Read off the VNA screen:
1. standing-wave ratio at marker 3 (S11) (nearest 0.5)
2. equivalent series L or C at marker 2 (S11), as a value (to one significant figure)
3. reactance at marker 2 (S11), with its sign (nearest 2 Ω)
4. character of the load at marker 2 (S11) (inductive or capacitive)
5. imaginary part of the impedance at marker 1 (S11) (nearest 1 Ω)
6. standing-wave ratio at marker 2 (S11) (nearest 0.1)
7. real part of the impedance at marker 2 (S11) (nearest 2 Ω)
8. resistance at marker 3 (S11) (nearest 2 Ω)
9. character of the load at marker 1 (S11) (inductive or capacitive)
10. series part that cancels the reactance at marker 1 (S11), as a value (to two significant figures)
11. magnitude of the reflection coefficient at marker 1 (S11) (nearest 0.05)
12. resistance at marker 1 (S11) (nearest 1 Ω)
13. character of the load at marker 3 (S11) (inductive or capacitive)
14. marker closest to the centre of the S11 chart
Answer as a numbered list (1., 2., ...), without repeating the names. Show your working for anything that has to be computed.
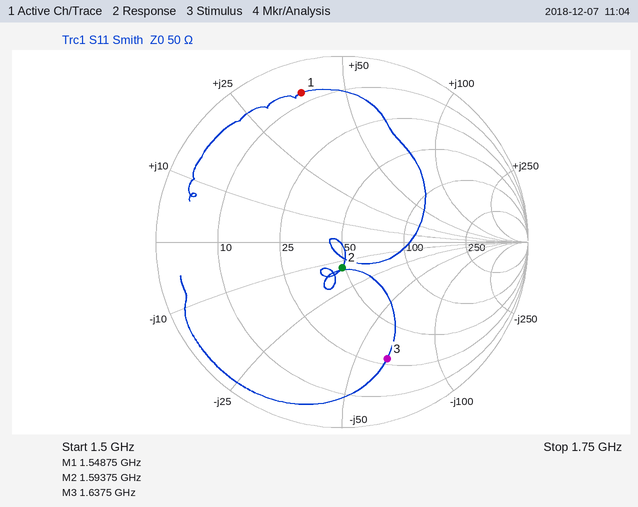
1. 5.0
2. C = 1/(2π × 1.59375 GHz × 14 Ω) ≈ 7 pF
3. -14 Ω
4. capacitive
5. +38 Ω
6. 1.3
7. 48 Ω
8. 28 Ω
9. inductive
10. C = 1/(2π × 1.54875 GHz × 38 Ω) ≈ 2.7 pF
11. 0.85
12. 7 Ω
13. capacitive
14. marker 2
